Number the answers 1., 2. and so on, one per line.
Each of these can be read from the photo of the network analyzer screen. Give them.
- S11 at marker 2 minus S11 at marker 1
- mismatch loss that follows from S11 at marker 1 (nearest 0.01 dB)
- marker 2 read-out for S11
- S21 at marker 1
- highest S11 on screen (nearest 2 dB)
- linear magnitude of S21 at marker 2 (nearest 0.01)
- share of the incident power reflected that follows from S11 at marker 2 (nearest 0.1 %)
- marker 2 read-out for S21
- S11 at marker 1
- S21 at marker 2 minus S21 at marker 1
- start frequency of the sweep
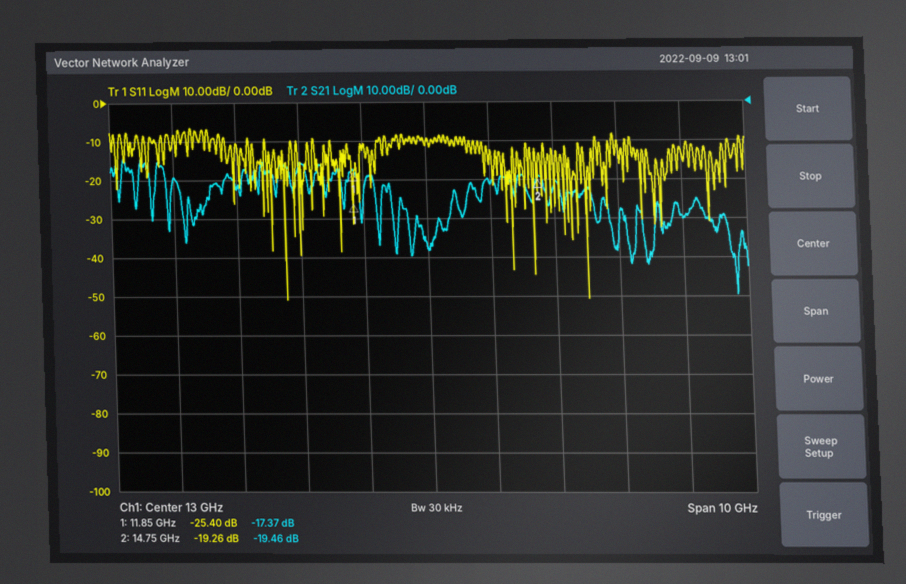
1. 6.14 dB
2. 0.01 dB
3. -19.26 dB
4. -17.37 dB
5. -6 dB
6. 0.11
7. 1.2 %
8. -19.46 dB
9. -25.40 dB
10. -2.09 dB
11. 8 GHz
